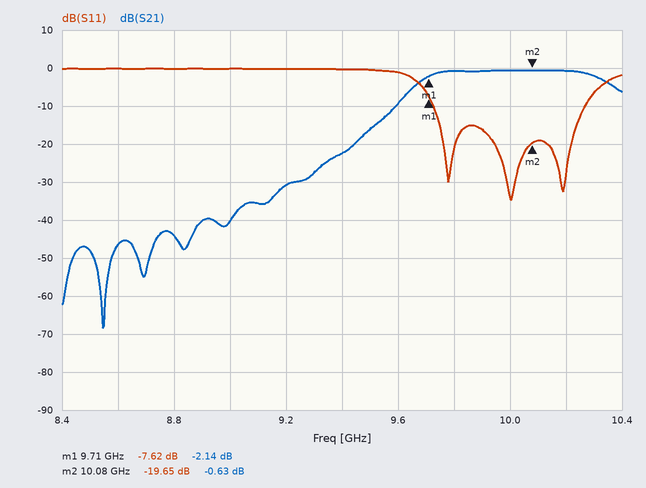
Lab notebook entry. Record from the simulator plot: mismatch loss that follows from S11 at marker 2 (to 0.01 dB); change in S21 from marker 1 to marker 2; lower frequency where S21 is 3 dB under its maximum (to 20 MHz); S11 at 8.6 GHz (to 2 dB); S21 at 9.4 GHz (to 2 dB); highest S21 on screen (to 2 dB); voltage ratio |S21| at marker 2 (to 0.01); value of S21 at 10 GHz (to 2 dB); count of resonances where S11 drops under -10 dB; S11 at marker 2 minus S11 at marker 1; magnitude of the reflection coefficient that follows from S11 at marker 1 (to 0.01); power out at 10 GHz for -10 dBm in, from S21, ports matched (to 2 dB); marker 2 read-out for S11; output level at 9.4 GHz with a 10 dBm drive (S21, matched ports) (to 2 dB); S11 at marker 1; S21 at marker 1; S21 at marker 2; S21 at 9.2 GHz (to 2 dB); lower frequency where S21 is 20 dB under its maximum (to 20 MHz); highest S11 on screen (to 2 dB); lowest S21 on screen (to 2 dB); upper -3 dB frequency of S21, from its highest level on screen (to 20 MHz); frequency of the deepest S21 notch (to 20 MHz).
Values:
0.05 dB
1.51 dB
9.68 GHz
0 dB
-22 dB
0 dB
0.93
0 dB
3
-12.03 dB
0.42
-10 dBm
-19.65 dB
-12 dBm
-7.62 dB
-2.14 dB
-0.63 dB
-30 dB
9.44 GHz
0 dB
-68 dB
10.34 GHz
8.54 GHz
